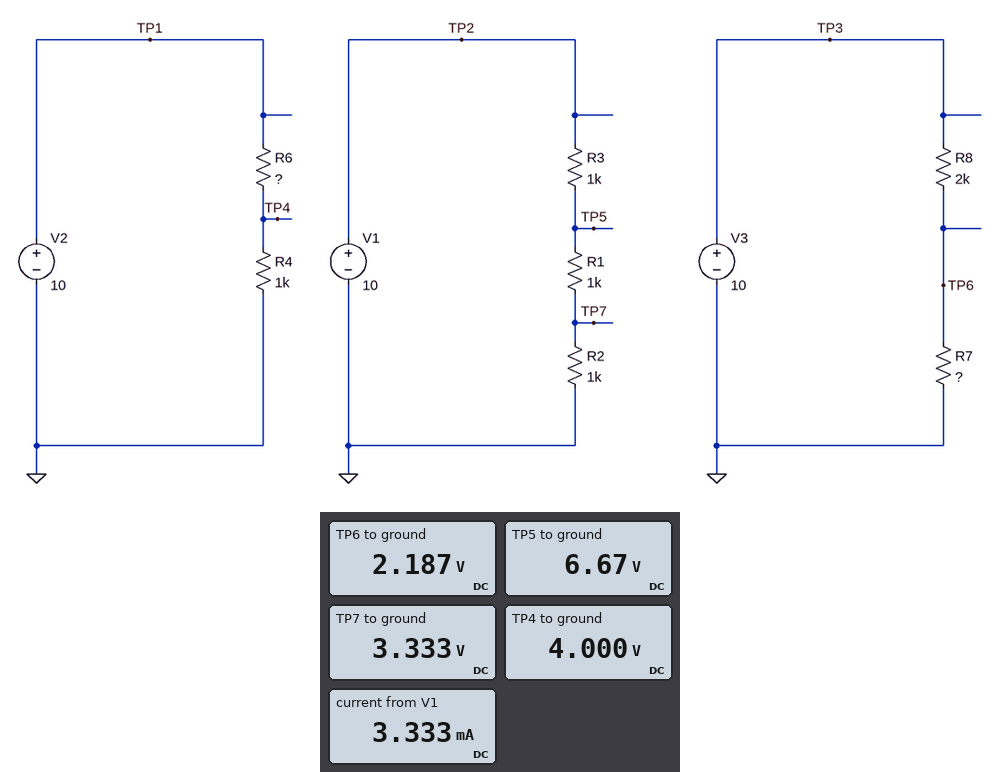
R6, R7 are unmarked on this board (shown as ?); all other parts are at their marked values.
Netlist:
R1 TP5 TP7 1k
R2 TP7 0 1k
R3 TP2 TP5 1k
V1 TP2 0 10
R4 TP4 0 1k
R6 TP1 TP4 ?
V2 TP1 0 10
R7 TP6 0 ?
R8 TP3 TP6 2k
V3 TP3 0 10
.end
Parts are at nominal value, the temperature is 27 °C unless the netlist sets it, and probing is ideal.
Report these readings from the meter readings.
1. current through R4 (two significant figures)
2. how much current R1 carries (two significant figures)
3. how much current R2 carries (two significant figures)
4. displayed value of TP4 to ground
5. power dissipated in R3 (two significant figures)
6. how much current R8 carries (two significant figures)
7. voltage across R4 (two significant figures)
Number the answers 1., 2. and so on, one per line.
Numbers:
1. 4.0 mA
2. 3.3 mA
3. 3.3 mA
4. 4.000 V
5. 11 mW
6. 3.9 mA
7. 4.0 V
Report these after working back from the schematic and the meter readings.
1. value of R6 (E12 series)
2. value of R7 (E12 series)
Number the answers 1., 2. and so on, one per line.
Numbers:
1. 1.5 kΩ
2. 560 Ω
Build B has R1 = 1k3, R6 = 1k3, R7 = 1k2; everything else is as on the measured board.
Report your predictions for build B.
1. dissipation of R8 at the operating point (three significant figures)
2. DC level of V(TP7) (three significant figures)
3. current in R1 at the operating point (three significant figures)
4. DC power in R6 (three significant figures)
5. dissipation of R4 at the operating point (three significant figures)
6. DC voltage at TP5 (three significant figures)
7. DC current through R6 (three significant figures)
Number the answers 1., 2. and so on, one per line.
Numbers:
1. 19.5 mW
2. 3.03 V
3. 3.03 mA
4. 24.6 mW
5. 18.9 mW
6. 6.97 V
7. 4.35 mA
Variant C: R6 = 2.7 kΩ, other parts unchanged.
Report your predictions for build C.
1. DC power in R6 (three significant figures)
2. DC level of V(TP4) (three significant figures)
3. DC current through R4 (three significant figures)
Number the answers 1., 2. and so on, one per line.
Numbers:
1. 19.7 mW
2. 2.70 V
3. 2.70 mA
